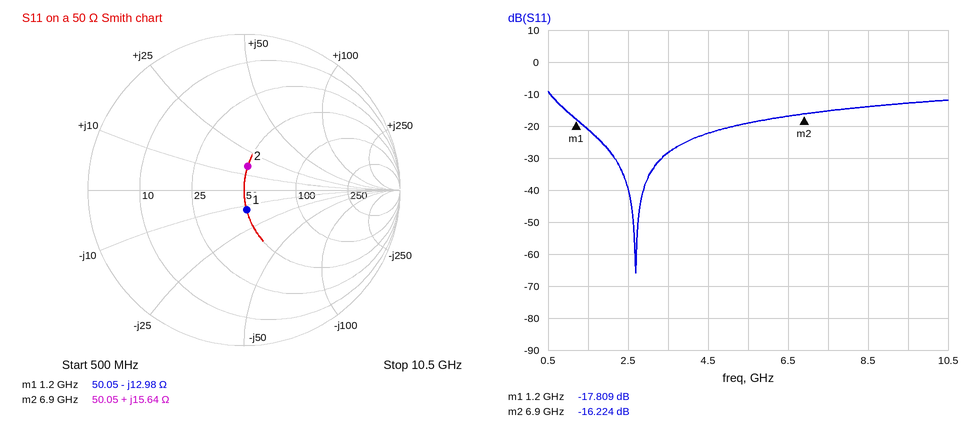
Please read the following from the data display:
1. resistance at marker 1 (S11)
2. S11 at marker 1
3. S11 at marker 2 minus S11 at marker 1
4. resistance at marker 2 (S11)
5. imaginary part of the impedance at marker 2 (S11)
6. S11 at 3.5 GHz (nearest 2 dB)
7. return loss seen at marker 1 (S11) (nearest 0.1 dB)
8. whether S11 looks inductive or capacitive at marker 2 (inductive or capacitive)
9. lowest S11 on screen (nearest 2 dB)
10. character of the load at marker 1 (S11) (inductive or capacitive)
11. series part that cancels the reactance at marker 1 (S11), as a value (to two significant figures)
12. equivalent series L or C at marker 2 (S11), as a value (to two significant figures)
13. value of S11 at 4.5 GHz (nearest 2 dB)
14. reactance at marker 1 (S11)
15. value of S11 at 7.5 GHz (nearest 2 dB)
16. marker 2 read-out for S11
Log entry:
50.05 Ω
-17.809 dB
1.585 dB
50.05 Ω
+15.64 Ω
-28 dB
17.8 dB
inductive
-66 dB
capacitive
1.7 nH
360 pH
-22 dB
-12.98 Ω
-16 dB
-16.224 dB
